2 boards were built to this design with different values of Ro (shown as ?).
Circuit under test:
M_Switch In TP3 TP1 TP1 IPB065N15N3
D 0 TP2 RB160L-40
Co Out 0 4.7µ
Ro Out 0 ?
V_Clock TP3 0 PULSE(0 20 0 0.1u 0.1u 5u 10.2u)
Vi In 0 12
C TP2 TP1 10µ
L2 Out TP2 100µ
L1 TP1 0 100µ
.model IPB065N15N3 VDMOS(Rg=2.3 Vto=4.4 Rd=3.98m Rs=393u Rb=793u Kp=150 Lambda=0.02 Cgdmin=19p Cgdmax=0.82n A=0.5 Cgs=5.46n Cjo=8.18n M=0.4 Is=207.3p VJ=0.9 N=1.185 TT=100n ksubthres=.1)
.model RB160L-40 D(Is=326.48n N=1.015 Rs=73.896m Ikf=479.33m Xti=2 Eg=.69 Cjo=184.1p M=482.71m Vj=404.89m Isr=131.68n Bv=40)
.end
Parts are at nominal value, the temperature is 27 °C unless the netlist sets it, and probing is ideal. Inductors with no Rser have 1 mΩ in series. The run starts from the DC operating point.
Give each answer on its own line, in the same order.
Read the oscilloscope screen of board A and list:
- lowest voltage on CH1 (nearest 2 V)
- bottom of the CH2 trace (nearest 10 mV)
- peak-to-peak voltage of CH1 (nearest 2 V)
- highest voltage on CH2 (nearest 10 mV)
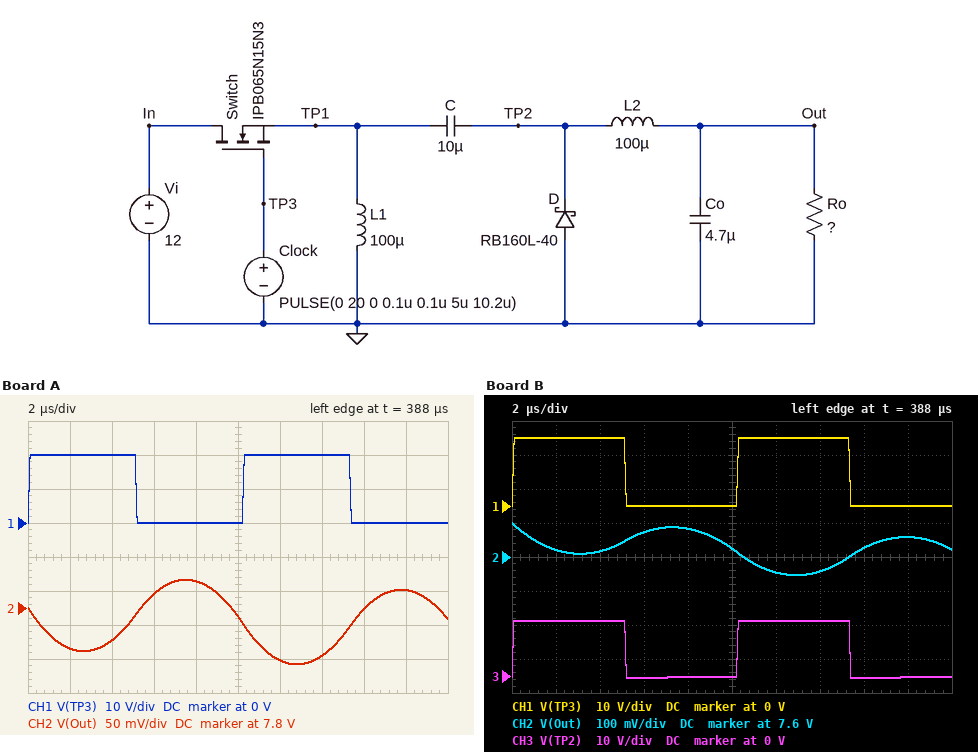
0 V
7.72 V
20 V
7.84 V
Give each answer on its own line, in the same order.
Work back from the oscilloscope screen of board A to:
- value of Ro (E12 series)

12 Ω
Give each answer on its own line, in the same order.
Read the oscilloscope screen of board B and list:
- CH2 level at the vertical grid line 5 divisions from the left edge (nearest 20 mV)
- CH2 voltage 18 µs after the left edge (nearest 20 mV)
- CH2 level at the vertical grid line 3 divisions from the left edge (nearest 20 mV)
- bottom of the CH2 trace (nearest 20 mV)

7.62 V
7.66 V
7.68 V
7.54 V
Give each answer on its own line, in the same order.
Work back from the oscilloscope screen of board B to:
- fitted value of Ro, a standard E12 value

27 Ω
